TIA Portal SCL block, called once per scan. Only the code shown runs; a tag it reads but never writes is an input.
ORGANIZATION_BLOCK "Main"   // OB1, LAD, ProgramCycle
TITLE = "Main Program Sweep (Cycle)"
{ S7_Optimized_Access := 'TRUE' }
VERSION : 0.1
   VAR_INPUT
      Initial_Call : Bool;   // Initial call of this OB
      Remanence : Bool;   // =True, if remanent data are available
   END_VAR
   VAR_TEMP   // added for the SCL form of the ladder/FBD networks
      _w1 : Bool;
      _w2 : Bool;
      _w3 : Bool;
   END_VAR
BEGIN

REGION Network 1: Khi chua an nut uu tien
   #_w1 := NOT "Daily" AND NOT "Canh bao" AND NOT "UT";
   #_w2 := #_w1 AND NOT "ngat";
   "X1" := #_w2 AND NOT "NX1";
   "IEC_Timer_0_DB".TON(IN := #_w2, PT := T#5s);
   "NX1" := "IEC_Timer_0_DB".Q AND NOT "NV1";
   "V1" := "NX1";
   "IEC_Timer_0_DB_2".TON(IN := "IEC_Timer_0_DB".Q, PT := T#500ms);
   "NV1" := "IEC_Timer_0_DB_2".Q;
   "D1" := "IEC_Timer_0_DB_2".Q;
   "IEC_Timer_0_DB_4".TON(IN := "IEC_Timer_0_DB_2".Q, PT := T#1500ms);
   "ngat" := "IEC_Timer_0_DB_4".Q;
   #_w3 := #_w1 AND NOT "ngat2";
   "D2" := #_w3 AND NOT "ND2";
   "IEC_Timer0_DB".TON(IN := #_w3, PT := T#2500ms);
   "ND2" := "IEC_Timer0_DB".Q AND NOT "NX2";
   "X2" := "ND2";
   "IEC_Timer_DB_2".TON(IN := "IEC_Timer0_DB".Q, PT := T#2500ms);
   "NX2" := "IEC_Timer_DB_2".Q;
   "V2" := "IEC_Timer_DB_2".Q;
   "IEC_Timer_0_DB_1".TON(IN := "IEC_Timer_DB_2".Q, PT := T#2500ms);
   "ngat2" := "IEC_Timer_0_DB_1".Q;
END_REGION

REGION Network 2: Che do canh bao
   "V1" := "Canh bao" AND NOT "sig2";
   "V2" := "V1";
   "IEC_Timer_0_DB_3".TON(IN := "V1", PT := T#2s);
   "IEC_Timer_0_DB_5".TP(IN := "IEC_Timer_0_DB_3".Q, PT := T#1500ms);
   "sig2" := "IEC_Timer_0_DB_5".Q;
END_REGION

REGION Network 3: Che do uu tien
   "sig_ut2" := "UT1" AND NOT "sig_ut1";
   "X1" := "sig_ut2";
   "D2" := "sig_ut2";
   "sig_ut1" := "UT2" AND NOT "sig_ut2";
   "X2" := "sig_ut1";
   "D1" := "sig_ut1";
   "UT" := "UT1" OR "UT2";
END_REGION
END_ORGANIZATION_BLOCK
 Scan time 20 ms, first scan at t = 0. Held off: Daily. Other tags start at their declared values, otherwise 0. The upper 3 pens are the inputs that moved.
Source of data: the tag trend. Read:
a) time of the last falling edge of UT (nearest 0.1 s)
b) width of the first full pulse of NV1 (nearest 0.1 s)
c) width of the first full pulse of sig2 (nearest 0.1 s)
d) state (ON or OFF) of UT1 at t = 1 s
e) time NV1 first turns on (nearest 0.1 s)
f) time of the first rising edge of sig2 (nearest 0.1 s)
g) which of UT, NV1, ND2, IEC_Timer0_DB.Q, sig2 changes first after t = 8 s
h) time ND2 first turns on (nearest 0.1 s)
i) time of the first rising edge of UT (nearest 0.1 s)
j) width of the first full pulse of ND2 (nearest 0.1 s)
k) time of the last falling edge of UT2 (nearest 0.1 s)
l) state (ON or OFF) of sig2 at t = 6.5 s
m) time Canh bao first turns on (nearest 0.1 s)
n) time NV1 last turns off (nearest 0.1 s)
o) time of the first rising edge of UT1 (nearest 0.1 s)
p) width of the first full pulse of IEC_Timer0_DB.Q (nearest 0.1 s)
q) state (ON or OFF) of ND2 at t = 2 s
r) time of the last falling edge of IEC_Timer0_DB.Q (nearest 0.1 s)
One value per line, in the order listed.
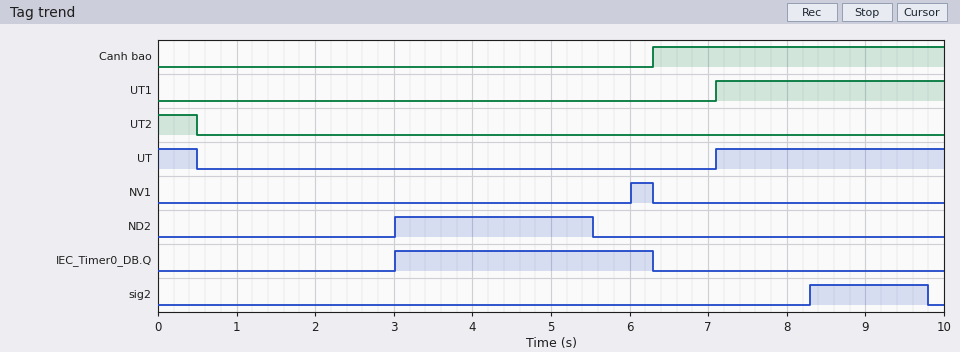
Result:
0.5 s
0.3 s
1.5 s
OFF
6.0 s
8.3 s
sig2
3.0 s
7.1 s
2.5 s
0.5 s
OFF
6.3 s
6.3 s
7.1 s
3.3 s
OFF
6.3 s
